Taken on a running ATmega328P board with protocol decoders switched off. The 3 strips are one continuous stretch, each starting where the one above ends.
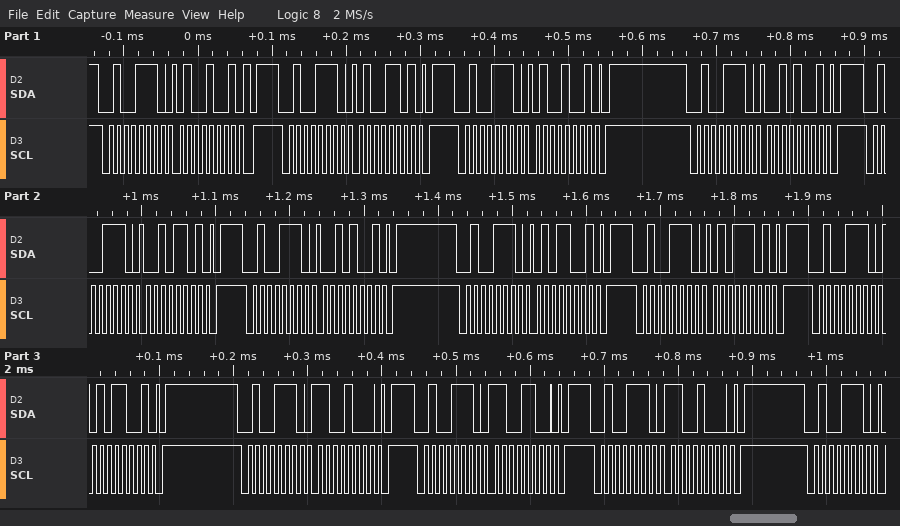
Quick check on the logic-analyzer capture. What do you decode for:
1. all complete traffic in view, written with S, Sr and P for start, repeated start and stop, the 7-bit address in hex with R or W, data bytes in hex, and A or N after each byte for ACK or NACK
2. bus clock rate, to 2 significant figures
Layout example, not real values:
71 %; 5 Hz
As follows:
S 27W A 49 A P S 27W A 4D A P S 27W A 49 A P S 27W A 29 A P S 27W A 2D A P S 27W A 29 A P S 27W A 59 A P S 27W A 5D A P S 27W A 59 A P S 27W A C8 A P S 27W A CC A P S 27W A C8 A P S 27W A; 100 kHz
